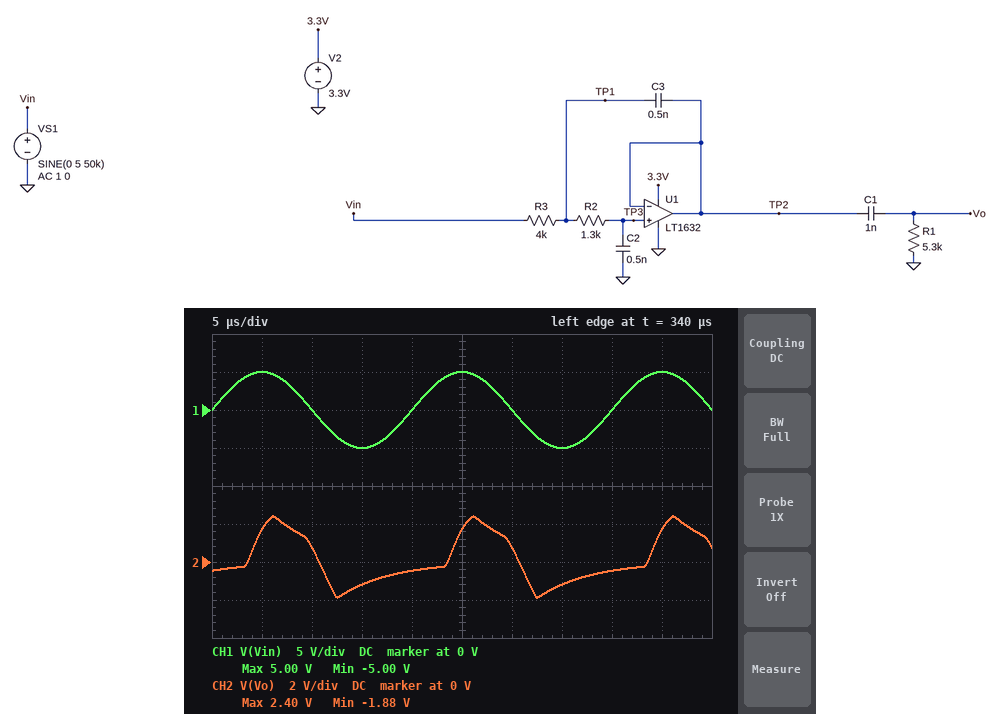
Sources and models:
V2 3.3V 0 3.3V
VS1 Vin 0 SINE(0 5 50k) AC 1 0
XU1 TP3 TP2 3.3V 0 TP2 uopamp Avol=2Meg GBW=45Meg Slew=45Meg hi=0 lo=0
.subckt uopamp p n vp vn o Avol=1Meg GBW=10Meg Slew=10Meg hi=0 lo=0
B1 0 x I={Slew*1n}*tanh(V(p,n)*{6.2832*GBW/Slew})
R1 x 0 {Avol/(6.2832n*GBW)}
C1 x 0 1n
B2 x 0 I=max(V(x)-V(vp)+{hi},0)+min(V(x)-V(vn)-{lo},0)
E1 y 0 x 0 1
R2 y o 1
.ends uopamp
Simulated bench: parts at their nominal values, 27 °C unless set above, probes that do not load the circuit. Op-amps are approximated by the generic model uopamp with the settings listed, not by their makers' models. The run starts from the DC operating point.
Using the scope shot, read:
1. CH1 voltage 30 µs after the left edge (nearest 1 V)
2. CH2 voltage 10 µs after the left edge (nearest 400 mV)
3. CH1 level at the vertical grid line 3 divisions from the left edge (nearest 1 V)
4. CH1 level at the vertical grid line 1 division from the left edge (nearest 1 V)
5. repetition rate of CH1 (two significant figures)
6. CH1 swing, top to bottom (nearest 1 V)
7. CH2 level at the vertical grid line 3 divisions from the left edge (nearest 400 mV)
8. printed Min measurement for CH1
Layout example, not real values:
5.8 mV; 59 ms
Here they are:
0 V; 800 mV; -5 V; 5 V; 50 kHz; 10 V; -1.2 V; -5.00 V
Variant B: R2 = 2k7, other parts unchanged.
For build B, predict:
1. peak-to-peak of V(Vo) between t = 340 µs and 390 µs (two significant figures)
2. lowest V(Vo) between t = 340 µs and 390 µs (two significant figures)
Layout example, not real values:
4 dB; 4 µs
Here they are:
4.0 V; -1.8 V
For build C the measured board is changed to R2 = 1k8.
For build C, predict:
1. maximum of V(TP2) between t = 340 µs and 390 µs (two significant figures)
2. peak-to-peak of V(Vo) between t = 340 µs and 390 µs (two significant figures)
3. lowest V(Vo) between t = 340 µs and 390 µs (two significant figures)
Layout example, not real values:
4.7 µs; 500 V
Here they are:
3.3 V; 4.2 V; -1.8 V
